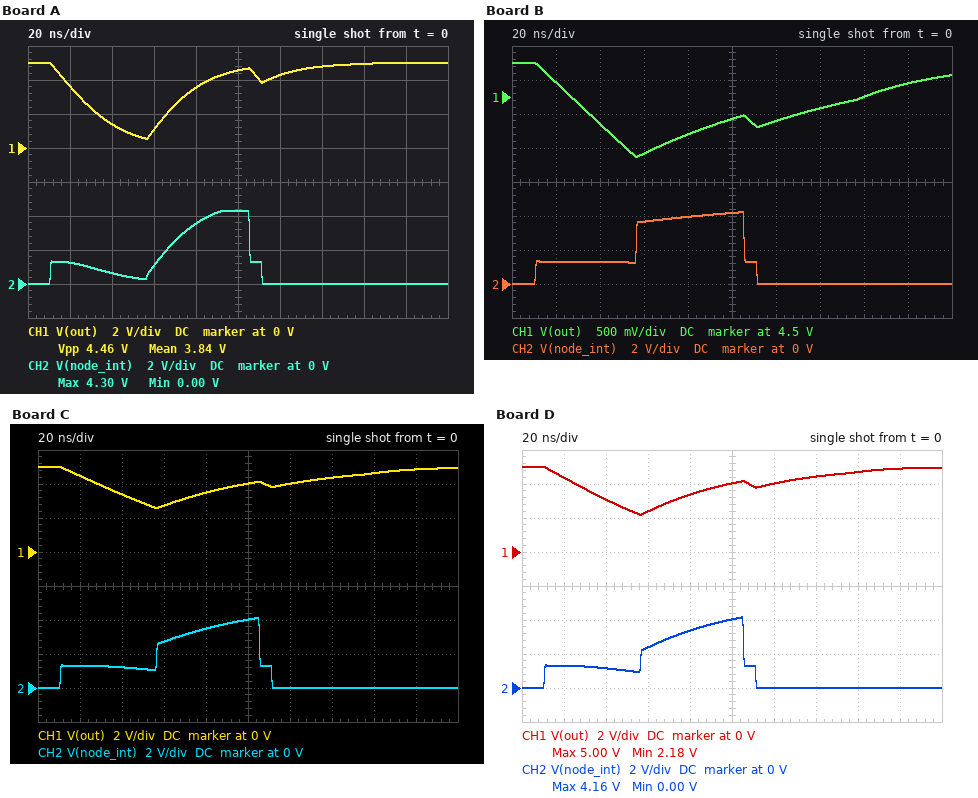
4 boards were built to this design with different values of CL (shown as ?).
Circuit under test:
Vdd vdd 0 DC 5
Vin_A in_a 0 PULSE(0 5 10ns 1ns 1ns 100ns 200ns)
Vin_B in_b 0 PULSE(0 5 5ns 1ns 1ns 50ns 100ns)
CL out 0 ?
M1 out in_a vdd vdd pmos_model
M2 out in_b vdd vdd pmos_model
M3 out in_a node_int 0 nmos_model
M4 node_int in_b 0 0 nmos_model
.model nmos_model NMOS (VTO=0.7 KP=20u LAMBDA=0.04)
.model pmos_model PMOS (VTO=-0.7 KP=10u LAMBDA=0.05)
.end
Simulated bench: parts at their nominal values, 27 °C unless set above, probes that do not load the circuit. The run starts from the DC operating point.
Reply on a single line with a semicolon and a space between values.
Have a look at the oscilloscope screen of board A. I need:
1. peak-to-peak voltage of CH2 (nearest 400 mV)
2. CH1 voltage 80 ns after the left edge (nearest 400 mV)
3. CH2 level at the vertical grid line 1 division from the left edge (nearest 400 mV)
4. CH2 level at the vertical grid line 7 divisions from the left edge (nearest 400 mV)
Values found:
4.4 V; 3.6 V; 1.2 V; 0 V
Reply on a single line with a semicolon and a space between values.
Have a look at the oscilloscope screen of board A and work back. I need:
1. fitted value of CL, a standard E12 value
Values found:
680 fF
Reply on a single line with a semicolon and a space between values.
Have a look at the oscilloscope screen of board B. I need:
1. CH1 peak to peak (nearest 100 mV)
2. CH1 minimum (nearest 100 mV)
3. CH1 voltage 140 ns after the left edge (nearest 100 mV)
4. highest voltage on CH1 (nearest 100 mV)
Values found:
1.4 V; 3.6 V; 4.3 V; 5.0 V
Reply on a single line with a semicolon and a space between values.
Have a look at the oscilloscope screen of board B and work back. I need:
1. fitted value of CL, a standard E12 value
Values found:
3.3 pF
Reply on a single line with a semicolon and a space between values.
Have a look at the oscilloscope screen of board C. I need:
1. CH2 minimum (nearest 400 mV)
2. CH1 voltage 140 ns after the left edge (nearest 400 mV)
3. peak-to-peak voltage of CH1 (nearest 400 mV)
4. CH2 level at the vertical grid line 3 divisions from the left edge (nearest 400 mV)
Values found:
0 V; 4.4 V; 2.4 V; 2.8 V
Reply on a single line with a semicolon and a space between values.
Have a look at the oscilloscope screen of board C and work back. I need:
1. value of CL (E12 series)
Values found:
1.8 pF
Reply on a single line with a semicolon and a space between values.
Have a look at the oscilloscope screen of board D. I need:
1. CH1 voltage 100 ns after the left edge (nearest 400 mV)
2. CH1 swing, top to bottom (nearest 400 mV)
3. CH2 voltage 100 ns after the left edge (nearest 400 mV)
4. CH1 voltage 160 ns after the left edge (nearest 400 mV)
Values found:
4.0 V; 2.8 V; 4.0 V; 4.8 V
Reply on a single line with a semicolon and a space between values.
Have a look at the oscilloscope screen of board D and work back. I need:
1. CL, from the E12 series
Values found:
1.5 pF
